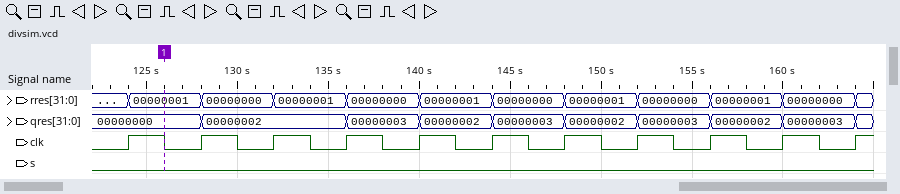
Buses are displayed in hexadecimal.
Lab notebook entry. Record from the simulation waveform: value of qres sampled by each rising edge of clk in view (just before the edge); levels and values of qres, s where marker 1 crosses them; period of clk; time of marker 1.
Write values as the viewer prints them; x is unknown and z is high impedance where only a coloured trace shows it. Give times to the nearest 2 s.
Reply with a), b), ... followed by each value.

a) 00000000, 00000000, 00000002, 00000002, 00000003, 00000002, 00000003, 00000002, 00000003, 00000002, 00000003
b) qres=00000000, s=0
c) 4 s
d) 126 s
